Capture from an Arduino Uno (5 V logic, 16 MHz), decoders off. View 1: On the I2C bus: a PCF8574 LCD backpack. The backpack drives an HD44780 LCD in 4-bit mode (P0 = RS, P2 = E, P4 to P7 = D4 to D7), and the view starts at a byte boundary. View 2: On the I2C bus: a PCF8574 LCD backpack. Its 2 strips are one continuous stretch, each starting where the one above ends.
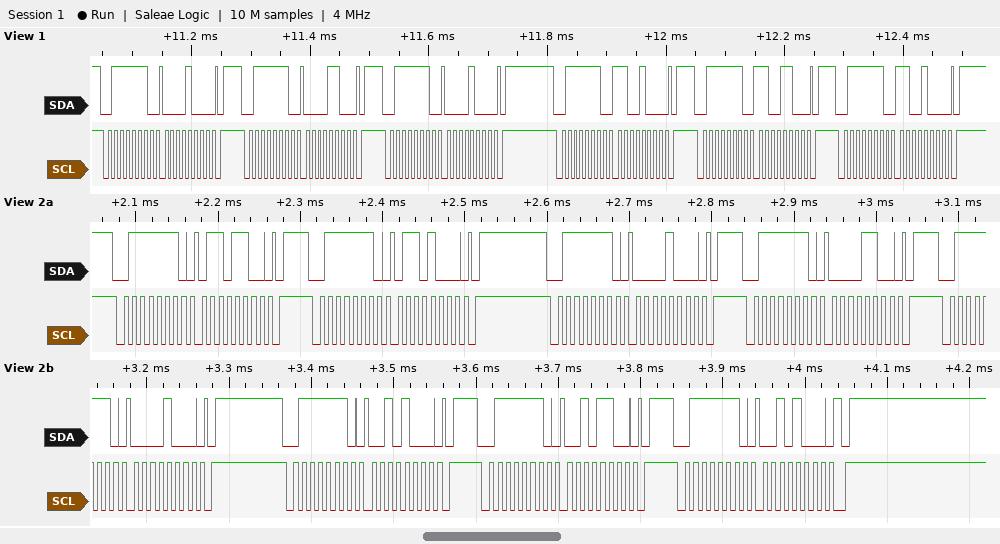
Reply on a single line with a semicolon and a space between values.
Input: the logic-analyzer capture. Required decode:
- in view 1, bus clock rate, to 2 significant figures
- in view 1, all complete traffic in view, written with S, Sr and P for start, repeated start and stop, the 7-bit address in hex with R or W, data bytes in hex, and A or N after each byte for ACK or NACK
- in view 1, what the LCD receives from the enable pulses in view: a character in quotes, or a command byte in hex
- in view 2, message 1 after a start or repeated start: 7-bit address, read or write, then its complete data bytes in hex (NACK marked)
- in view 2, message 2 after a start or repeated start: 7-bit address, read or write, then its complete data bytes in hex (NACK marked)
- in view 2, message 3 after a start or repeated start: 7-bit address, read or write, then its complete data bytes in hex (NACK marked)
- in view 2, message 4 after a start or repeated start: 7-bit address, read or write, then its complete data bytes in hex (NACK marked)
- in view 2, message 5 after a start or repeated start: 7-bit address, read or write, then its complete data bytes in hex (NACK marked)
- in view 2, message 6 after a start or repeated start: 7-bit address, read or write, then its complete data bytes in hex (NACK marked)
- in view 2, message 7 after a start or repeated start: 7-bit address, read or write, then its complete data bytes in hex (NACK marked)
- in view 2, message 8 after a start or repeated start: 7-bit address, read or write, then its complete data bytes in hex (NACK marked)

100 kHz; S 3FW A 08 A P S 3FW A 0C A P S 3FW A 08 A P S 3FW A C8 A P S 3FW A CC A P S 3FW A C8 A P; 0x0C; 0x3F write: 6C; 0x3F write: 68; 0x3F write: 08; 0x3F write: 0C; 0x3F write: 08; 0x3F write: 28; 0x3F write: 2C; 0x3F write: 28
